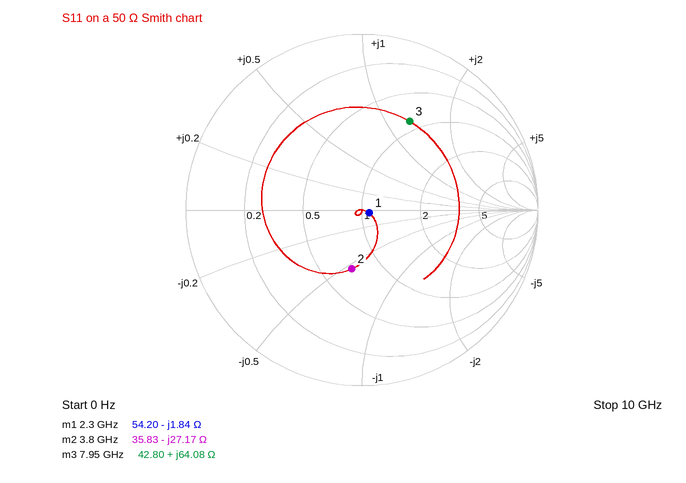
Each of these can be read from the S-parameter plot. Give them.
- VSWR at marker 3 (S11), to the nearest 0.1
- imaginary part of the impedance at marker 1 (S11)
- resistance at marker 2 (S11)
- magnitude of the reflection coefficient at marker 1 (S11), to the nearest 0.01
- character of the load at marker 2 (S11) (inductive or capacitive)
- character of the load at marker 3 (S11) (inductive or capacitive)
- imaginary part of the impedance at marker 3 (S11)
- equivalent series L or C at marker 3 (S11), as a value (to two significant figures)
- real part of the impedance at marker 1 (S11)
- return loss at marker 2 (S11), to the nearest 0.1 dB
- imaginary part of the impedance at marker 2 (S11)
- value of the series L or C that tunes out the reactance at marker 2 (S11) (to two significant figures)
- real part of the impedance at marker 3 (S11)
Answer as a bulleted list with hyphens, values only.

- 3.7
- -1.84 Ω
- 35.83 Ω
- 0.04
- capacitive
- inductive
- +64.08 Ω
- 1.3 nH
- 54.20 Ω
- 9.4 dB
- -27.17 Ω
- 1.1 nH
- 42.80 Ω
